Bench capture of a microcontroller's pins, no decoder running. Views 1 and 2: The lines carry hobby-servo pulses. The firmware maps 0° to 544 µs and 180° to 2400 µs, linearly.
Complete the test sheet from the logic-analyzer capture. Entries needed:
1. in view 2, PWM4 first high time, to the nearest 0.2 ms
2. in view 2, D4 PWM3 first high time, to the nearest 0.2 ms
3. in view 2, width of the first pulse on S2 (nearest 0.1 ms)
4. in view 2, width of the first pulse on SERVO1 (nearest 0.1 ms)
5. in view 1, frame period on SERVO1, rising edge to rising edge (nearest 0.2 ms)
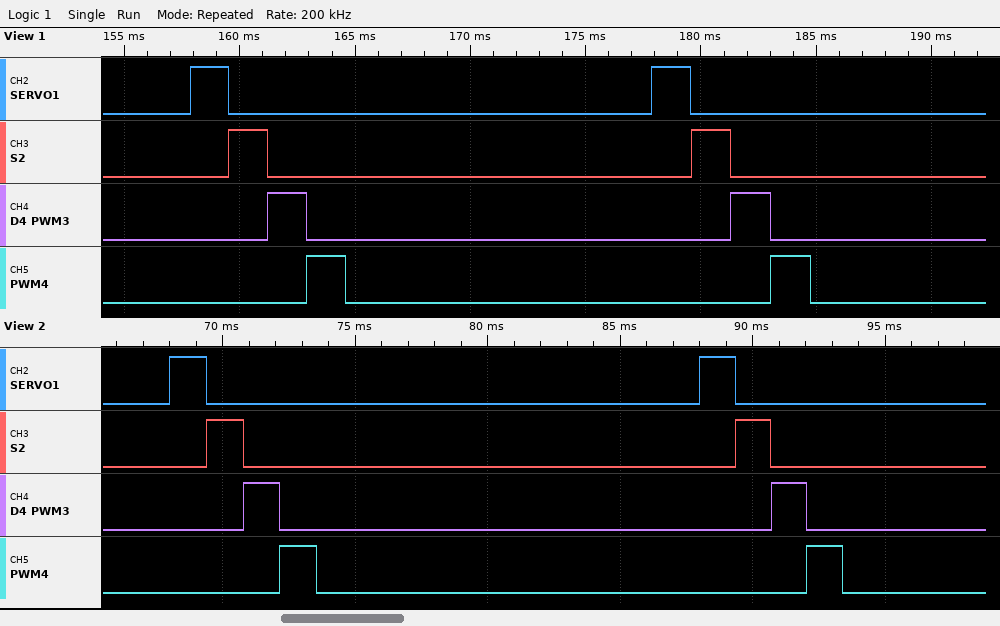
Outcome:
1.4 ms
1.4 ms
1.4 ms
1.4 ms
20.0 ms
